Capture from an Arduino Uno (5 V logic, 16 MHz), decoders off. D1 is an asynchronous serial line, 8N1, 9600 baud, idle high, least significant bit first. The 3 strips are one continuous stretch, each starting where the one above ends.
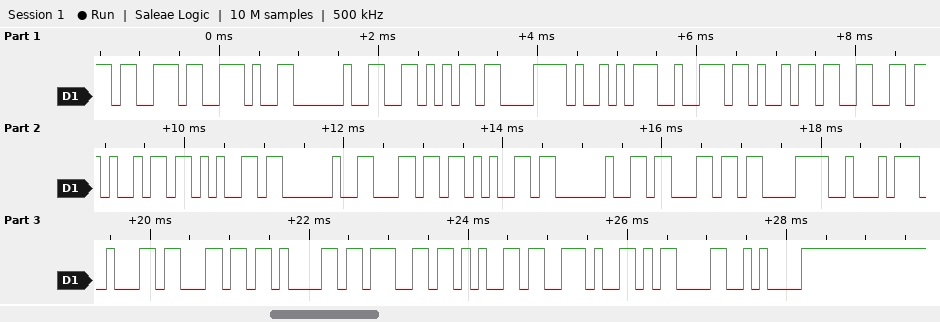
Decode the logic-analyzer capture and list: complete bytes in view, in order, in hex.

73 2E 20 56 C3 A9 72 69 66 69 65 20 6C 65 20 63 C3 A2 62 6C 61 67 65 2E 0D 0A
